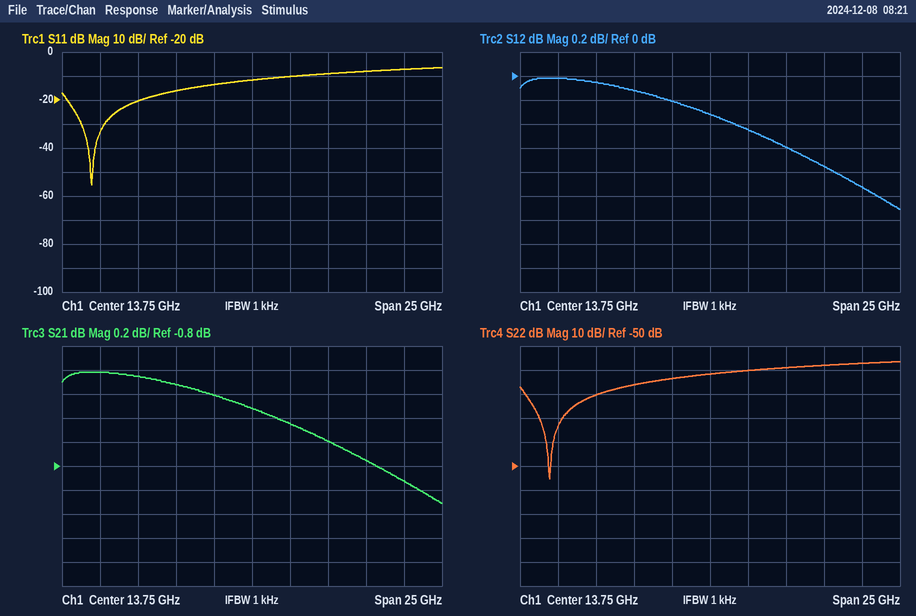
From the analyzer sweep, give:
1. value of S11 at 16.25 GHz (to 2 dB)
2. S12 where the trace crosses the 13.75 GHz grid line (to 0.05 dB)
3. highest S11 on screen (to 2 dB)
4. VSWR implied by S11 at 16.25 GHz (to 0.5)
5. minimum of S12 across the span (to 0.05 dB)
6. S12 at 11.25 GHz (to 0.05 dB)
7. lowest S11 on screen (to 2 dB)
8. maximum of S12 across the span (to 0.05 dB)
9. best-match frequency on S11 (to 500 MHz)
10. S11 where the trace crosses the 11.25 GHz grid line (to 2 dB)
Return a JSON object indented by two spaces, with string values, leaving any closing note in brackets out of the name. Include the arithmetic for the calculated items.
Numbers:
{
  "value of S11 at 16.25 GHz": "-10 dB",
  "S12 where the trace crosses the 13.75 GHz grid line": "-0.30 dB",
  "highest S11 on screen": "-6 dB",
  "VSWR implied by S11 at 16.25 GHz": "|Γ| = 10^(-10/20) = 0.3162; VSWR = (1 + 0.3162)/(1 − 0.3162) ≈ 1.92, so 2.0 to the nearest 0.5",
  "minimum of S12 across the span": "-1.10 dB",
  "S12 at 11.25 GHz": "-0.20 dB",
  "lowest S11 on screen": "-56 dB",
  "maximum of S12 across the span": "0.00 dB",
  "best-match frequency on S11": "3.0 GHz",
  "S11 where the trace crosses the 11.25 GHz grid line": "-14 dB"
}
